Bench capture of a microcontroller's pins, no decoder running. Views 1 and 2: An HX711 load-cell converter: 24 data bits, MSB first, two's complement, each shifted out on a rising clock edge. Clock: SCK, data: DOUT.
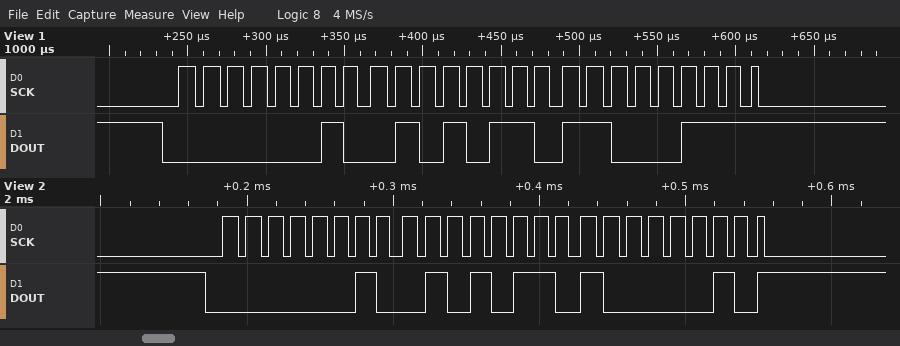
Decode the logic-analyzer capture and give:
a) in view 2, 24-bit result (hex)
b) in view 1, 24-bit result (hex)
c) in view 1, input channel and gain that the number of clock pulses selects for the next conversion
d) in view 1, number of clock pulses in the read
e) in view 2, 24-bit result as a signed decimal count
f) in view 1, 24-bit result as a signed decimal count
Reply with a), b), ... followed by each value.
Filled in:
a) 0x025682
b) 0x0256C7
c) channel A, gain 128
d) 25
e) 153218
f) 153287
